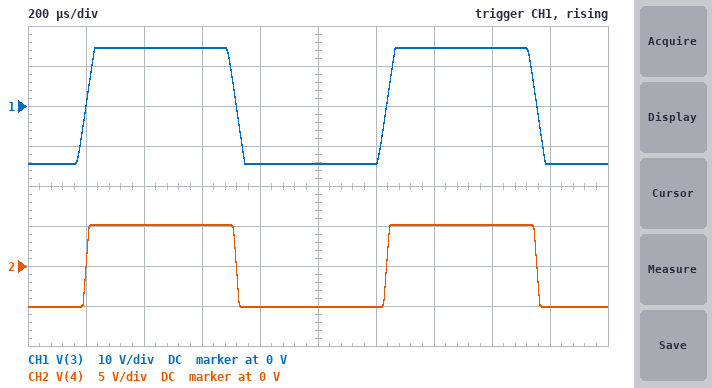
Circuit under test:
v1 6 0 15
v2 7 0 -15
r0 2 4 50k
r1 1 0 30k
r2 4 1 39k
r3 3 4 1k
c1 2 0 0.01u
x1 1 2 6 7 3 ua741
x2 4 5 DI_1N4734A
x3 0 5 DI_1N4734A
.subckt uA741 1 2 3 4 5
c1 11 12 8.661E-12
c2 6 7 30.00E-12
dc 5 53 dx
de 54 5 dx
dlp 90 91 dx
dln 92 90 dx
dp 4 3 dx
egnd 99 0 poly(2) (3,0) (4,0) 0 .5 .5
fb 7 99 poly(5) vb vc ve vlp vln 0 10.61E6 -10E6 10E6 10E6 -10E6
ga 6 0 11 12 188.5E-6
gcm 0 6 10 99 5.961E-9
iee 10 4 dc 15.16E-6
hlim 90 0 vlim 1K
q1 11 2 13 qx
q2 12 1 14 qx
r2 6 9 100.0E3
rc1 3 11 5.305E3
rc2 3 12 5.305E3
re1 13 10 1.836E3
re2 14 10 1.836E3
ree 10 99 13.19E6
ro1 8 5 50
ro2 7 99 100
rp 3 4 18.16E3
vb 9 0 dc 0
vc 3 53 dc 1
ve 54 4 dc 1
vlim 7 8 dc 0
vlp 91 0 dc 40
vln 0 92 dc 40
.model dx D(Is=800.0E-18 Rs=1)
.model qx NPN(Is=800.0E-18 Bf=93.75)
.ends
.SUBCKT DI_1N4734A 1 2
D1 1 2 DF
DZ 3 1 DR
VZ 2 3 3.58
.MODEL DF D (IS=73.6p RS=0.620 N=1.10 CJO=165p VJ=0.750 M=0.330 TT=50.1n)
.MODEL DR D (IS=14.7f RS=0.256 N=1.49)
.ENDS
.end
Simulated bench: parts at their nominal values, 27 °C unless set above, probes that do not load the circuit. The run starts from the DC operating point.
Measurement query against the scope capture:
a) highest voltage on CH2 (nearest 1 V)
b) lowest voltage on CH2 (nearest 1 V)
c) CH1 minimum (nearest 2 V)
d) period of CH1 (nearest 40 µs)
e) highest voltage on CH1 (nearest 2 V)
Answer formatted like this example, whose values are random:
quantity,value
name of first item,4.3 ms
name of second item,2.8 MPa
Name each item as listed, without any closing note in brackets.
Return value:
quantity,value
highest voltage on CH2,5 V
lowest voltage on CH2,-5 V
CH1 minimum,-14 V
period of CH1,1.04 ms
highest voltage on CH1,14 V
